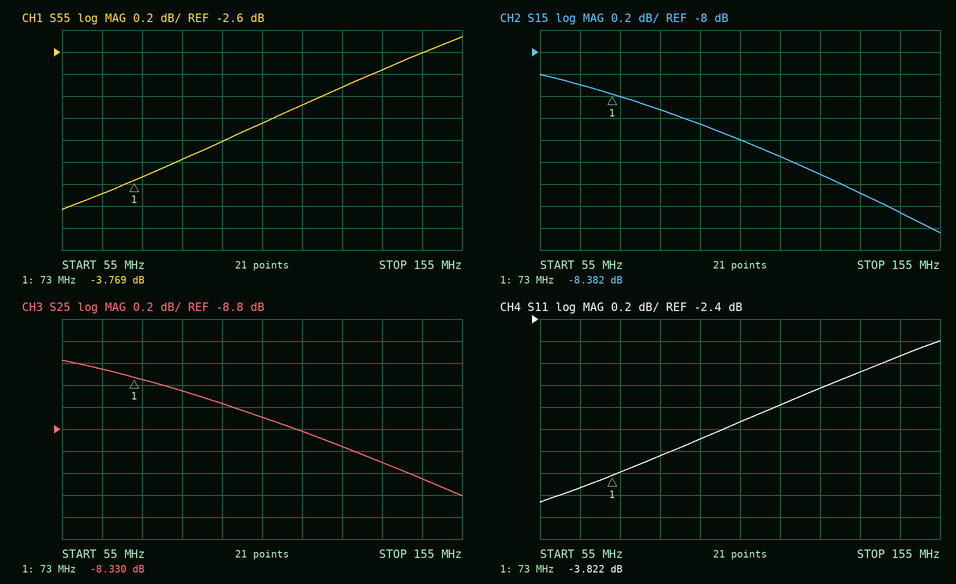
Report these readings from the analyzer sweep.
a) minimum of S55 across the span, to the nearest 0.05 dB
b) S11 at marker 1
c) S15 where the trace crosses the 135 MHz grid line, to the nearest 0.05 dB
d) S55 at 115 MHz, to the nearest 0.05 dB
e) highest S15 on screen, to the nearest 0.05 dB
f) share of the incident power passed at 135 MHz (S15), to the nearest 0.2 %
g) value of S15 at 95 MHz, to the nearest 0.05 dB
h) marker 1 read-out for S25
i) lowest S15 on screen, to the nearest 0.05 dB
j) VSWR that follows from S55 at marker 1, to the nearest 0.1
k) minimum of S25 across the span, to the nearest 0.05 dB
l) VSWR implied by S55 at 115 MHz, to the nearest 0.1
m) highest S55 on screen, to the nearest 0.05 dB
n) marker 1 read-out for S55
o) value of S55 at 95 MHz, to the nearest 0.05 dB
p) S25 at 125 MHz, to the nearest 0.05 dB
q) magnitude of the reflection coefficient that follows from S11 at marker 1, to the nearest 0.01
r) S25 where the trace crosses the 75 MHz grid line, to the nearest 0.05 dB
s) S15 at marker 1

-4.05 dB
-3.822 dB
-9.30 dB
-3.10 dB
-8.20 dB
11.8 %
-8.65 dB
-8.330 dB
-9.65 dB
4.7
-9.40 dB
5.7
-2.45 dB
-3.769 dB
-3.40 dB
-8.95 dB
0.64
-8.35 dB
-8.382 dB
